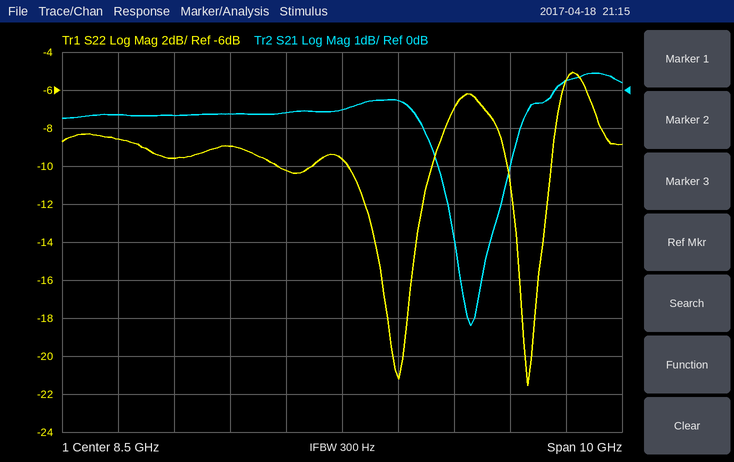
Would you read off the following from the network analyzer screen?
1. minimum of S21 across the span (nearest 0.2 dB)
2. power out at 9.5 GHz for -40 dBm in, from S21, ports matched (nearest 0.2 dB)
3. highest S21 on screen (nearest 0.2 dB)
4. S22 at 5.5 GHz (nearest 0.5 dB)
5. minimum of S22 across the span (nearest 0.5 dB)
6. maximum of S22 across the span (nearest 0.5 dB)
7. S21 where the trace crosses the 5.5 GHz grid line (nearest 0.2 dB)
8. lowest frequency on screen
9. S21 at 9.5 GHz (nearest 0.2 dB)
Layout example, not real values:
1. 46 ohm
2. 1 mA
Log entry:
1. -6.2 dB
2. -40.2 dBm
3. 0.4 dB
4. -9.5 dB
5. -21.5 dB
6. -5.0 dB
7. -0.6 dB
8. 3.5 GHz
9. -0.2 dB
